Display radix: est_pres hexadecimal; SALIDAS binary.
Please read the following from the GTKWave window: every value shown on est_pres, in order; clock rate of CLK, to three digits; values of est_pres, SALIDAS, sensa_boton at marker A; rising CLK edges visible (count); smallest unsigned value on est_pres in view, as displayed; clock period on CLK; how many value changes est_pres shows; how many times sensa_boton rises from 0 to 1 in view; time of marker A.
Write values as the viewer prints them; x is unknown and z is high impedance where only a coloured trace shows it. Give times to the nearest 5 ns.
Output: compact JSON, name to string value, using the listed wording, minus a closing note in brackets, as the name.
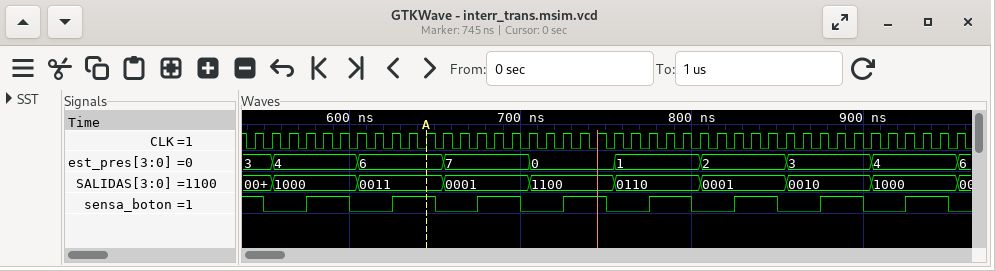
{"every value shown on est_pres, in order": "3, 4, 6, 7, 0, 1, 2, 3, 4, 6", "clock rate of CLK, to three digits": "100 MHz", "values of est_pres, SALIDAS, sensa_boton at marker A": "est_pres=6, SALIDAS=0011, sensa_boton=1", "rising CLK edges visible": "42", "smallest unsigned value on est_pres in view, as displayed": "0", "clock period on CLK": "10 ns", "how many value changes est_pres shows": "9", "how many times sensa_boton rises from 0 to 1 in view": "8", "time of marker A": "645 ns"}
